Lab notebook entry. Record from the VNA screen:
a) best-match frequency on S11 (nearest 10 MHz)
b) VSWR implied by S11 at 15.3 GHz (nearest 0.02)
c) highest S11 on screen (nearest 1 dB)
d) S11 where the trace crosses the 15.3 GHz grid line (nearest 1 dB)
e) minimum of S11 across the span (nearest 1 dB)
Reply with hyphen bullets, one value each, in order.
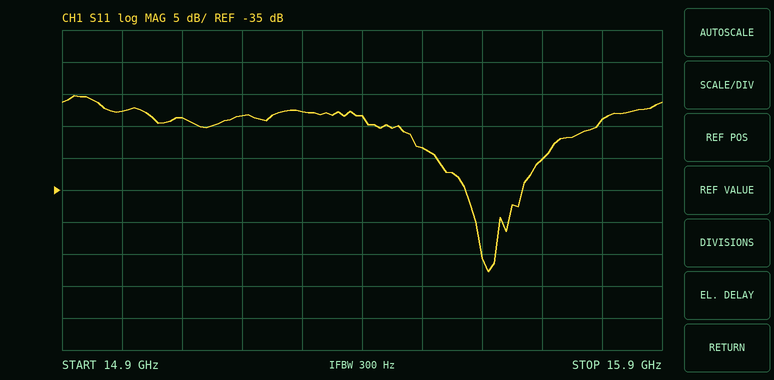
- 15.61 GHz
- 1.16
- -20 dB
- -23 dB
- -48 dB
